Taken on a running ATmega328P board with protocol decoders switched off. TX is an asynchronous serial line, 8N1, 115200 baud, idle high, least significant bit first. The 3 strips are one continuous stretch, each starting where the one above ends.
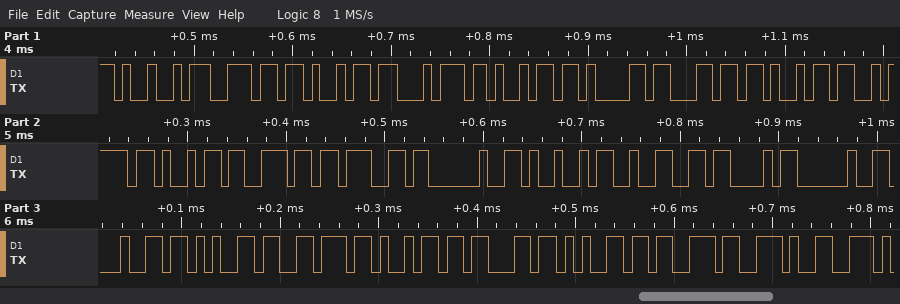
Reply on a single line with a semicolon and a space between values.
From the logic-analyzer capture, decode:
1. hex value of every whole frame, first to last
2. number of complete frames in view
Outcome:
49 6E 69 74 69 61 6C 69 7A 69 6E 67 20 49 32 43 20 64 65 76 69 63 65 73 2E; 25
